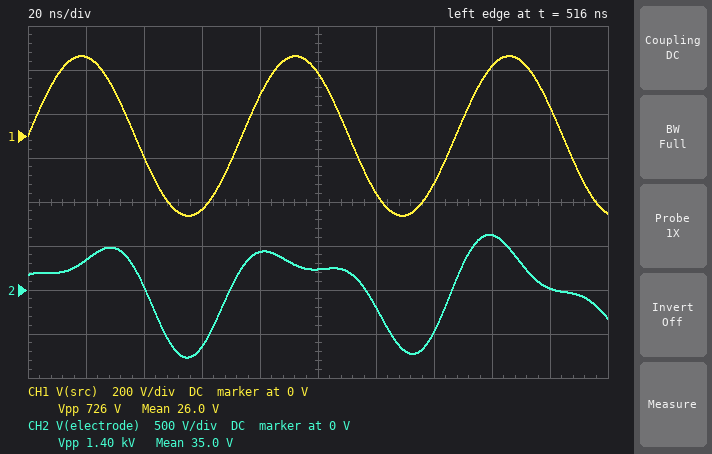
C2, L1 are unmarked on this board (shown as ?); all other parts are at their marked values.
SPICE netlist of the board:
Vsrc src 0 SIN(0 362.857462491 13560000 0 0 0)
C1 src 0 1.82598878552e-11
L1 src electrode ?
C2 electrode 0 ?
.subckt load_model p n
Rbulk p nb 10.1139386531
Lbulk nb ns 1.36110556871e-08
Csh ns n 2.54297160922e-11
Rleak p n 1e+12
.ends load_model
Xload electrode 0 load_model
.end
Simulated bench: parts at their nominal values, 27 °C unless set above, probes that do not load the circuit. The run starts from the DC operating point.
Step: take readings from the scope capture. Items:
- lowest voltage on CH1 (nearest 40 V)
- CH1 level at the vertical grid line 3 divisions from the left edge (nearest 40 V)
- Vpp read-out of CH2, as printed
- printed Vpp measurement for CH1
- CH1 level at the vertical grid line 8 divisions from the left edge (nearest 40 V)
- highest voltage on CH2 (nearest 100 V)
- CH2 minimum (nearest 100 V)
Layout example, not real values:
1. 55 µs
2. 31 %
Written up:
1. -360 V
2. -320 V
3. 1.40 kV
4. 726 V
5. 320 V
6. 600 V
7. -800 V
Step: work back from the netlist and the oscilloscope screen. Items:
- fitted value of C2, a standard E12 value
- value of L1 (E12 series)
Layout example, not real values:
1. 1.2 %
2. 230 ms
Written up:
1. 470 pF
2. 82 nH
